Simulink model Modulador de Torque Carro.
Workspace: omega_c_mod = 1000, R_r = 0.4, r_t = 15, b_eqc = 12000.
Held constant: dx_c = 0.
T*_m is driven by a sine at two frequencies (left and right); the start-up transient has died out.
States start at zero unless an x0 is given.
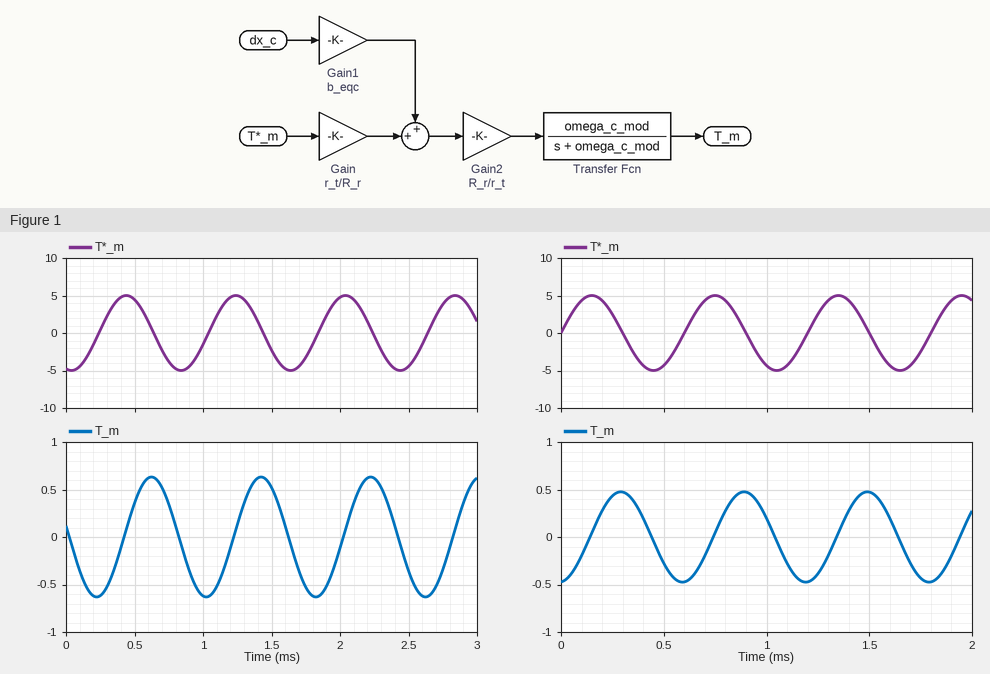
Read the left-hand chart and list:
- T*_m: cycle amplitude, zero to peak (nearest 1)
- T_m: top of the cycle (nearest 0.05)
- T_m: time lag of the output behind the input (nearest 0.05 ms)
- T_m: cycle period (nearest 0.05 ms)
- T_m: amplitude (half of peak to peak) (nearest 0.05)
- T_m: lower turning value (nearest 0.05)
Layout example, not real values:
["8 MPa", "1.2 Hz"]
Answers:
["5", "0.65", "0.20 ms", "0.80 ms", "0.65", "-0.65"]
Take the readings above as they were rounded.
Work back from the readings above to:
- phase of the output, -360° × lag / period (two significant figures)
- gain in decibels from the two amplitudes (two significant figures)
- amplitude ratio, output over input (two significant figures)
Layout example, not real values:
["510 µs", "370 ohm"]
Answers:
["-90°", "-18 dB", "0.13"]
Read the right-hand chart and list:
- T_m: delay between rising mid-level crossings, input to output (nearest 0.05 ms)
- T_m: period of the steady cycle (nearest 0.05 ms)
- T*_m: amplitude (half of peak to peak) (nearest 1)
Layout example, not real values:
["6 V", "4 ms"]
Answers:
["0.15 ms", "0.60 ms", "5"]
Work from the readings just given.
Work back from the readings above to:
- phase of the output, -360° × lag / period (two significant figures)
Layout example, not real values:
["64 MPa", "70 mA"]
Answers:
["-90°"]
